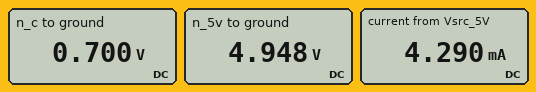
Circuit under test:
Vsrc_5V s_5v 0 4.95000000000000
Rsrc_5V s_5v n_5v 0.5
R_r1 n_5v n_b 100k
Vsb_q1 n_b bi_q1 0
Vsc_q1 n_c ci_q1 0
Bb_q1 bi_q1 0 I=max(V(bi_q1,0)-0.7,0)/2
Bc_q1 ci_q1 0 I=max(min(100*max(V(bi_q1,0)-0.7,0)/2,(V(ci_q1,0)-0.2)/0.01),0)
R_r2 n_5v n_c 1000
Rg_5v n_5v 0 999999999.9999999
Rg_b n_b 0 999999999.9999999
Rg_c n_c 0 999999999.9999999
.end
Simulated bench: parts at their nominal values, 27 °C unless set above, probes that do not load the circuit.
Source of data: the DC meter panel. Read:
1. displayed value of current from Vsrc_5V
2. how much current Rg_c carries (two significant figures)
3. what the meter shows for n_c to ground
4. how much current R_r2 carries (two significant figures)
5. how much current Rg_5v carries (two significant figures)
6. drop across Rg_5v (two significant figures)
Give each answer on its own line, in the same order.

4.290 mA
700 pA
0.700 V
4.2 mA
4.9 nA
4.9 V
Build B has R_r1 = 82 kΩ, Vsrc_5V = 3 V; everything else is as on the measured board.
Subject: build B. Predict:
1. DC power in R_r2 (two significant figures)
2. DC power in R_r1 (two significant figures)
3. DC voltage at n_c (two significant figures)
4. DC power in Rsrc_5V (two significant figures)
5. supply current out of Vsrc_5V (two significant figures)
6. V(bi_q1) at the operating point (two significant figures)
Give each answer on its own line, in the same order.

7.8 mW
64 µW
200 mV
4.0 µW
2.8 mA
700 mV
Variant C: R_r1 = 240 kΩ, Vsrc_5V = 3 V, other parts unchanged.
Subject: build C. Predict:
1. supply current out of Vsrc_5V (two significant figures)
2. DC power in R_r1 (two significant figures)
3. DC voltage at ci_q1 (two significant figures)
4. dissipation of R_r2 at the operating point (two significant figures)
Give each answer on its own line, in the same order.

970 µA
22 µW
2.0 V
920 µW
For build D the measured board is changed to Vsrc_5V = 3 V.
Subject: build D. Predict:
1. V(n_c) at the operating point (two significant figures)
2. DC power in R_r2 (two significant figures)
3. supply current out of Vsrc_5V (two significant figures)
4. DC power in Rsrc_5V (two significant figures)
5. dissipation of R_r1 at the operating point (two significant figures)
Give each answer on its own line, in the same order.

700 mV
5.3 mW
2.3 mA
2.7 µW
53 µW
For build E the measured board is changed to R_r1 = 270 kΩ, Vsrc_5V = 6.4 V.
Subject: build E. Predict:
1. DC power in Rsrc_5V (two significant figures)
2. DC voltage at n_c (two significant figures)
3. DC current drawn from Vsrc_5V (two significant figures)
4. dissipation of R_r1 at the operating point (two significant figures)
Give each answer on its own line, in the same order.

2.3 µW
4.3 V
2.1 mA
120 µW
